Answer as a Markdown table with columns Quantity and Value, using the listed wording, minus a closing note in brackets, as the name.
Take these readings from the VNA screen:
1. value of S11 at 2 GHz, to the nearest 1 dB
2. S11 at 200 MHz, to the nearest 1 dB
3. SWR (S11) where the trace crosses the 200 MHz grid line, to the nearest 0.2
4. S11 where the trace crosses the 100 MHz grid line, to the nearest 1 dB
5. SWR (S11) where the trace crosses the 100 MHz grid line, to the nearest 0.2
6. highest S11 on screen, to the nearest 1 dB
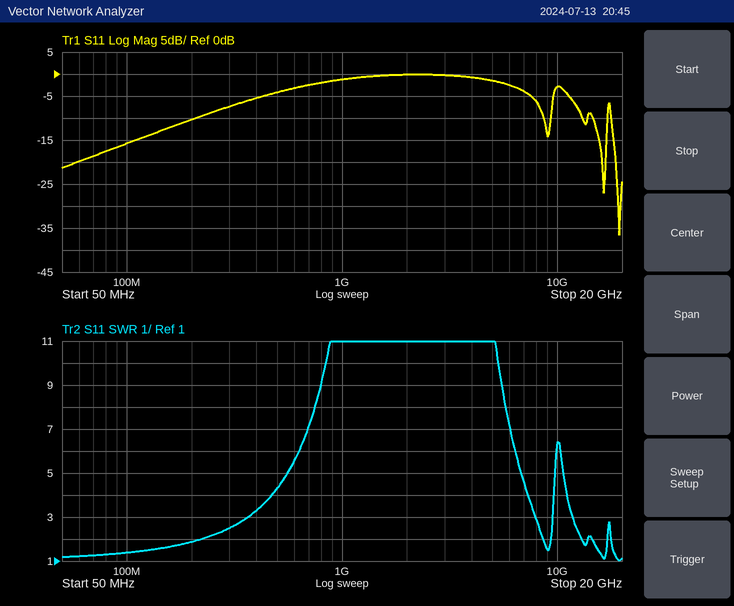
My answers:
| Quantity | Value |
|---|---|
| value of S11 at 2 GHz, to the nearest 1 dB | 0 dB |
| S11 at 200 MHz, to the nearest 1 dB | -10 dB |
| SWR (S11) where the trace crosses the 200 MHz grid line, to the nearest 0.2 | 1.8 |
| S11 where the trace crosses the 100 MHz grid line, to the nearest 1 dB | -16 dB |
| SWR (S11) where the trace crosses the 100 MHz grid line, to the nearest 0.2 | 1.4 |
| highest S11 on screen, to the nearest 1 dB | 0 dB |
